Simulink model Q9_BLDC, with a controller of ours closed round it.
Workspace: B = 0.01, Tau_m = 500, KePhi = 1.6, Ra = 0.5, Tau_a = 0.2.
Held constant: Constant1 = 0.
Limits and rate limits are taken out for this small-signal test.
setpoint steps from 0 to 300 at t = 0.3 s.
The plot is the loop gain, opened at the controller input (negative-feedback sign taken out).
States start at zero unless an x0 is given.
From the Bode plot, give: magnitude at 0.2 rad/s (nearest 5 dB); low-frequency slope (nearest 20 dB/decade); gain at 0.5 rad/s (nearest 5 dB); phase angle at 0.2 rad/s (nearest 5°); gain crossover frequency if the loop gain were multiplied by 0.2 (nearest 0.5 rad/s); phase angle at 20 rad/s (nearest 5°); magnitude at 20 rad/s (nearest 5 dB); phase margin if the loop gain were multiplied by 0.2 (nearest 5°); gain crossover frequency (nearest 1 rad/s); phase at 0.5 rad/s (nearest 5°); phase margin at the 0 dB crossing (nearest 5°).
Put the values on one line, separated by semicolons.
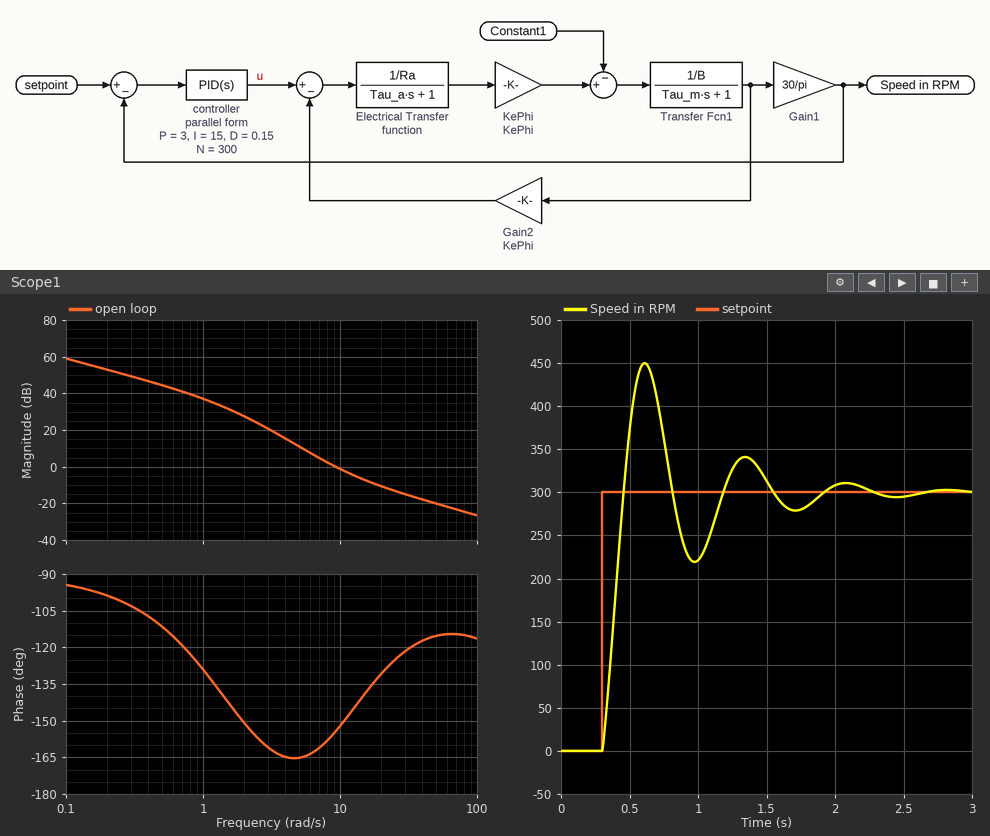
55 dB; -20 dB/decade; 45 dB; -100°; 4.5 rad/s; -130°; -10 dB; 15°; 9 rad/s; -110°; 25°
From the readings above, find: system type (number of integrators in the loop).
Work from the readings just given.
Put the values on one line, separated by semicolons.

1
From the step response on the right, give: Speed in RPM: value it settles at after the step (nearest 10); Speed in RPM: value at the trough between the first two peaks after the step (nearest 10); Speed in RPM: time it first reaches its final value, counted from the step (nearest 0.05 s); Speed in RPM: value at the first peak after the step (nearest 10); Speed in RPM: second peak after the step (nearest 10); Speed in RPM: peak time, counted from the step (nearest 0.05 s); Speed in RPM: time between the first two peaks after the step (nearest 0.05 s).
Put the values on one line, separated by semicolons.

300; 220; 0.15 s; 450; 340; 0.30 s; 0.75 s
